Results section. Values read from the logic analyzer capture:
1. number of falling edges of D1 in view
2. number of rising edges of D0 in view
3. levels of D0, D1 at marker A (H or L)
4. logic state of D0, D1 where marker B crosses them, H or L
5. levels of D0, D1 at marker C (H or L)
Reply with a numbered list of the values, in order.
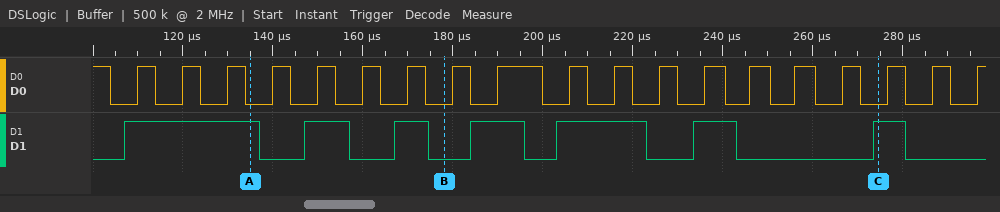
1. 7
2. 19
3. D0=L, D1=H
4. D0=L, D1=L
5. D0=L, D1=H
